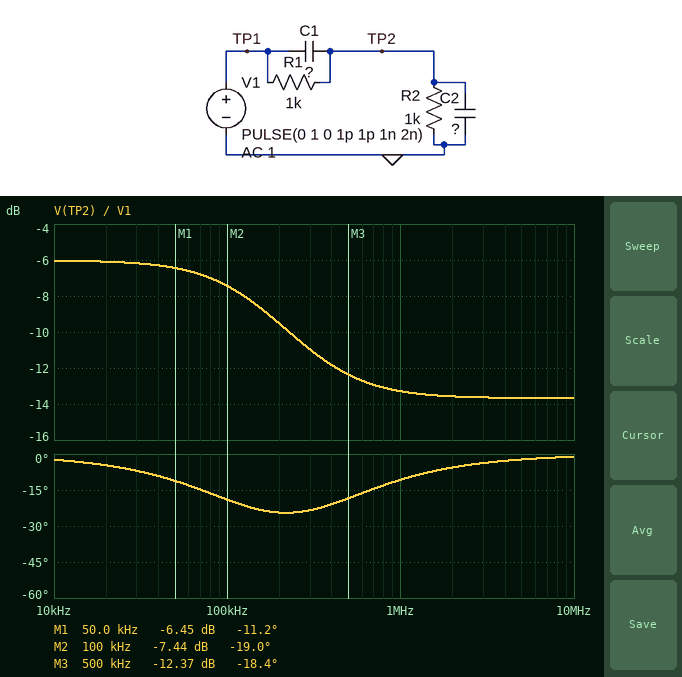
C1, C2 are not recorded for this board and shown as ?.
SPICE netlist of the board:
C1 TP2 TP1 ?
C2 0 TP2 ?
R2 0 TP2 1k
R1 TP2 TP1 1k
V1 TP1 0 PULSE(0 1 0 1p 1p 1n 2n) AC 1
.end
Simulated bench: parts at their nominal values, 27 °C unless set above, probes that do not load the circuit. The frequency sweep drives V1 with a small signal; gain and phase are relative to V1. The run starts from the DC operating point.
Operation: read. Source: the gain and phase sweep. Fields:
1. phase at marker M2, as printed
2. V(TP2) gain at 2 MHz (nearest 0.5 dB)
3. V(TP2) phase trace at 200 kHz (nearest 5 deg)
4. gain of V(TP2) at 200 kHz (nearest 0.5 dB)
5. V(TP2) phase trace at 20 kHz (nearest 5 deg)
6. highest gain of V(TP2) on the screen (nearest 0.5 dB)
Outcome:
-19.0 deg
-13.5 dB
-25 deg
-9.5 dB
-5 deg
-6.0 dB
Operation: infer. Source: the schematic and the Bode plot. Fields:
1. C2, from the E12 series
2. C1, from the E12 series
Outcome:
1.8 nF
470 pF
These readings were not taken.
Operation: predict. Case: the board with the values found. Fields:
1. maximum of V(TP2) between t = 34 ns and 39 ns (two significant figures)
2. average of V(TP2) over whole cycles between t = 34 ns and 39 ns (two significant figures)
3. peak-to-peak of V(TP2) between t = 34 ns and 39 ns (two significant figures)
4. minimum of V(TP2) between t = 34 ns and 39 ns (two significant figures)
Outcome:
210 mV
110 mV
210 mV
4.3 mV
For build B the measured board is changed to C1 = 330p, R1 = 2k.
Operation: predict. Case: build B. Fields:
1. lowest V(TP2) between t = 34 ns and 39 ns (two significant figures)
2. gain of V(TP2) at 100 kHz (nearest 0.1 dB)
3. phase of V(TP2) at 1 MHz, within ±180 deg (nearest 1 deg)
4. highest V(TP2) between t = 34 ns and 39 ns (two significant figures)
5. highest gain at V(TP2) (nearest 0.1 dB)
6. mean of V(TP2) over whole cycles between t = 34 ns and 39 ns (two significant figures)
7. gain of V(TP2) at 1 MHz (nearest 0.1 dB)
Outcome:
2.1 mV
-11.4 dB
-7 deg
160 mV
-9.5 dB
80 mV
-16.0 dB
